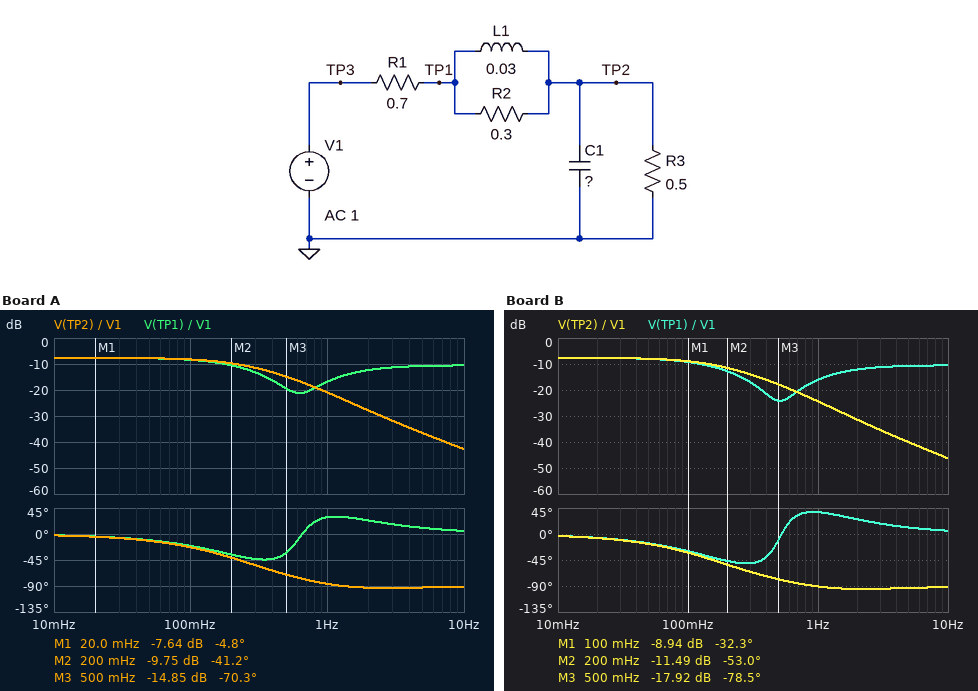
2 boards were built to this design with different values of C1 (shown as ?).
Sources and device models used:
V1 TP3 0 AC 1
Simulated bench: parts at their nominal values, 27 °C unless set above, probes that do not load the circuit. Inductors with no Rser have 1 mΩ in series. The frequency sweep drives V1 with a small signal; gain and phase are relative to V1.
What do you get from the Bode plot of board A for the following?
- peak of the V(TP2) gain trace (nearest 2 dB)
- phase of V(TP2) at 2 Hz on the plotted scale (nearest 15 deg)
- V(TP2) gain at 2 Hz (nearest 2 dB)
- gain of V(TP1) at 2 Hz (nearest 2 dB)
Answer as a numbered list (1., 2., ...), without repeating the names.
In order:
1. -8 dB
2. -90 deg
3. -28 dB
4. -12 dB
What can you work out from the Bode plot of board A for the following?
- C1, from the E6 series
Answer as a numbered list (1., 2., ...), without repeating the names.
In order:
1. 2.2 F
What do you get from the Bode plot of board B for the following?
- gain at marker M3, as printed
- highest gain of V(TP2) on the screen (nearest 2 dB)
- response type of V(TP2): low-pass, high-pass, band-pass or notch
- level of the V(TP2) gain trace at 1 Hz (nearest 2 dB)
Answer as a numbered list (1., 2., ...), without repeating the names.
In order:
1. -17.92 dB
2. -8 dB
3. low-pass
4. -24 dB
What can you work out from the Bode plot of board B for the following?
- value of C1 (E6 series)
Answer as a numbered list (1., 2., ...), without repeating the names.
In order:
1. 3.3 F
